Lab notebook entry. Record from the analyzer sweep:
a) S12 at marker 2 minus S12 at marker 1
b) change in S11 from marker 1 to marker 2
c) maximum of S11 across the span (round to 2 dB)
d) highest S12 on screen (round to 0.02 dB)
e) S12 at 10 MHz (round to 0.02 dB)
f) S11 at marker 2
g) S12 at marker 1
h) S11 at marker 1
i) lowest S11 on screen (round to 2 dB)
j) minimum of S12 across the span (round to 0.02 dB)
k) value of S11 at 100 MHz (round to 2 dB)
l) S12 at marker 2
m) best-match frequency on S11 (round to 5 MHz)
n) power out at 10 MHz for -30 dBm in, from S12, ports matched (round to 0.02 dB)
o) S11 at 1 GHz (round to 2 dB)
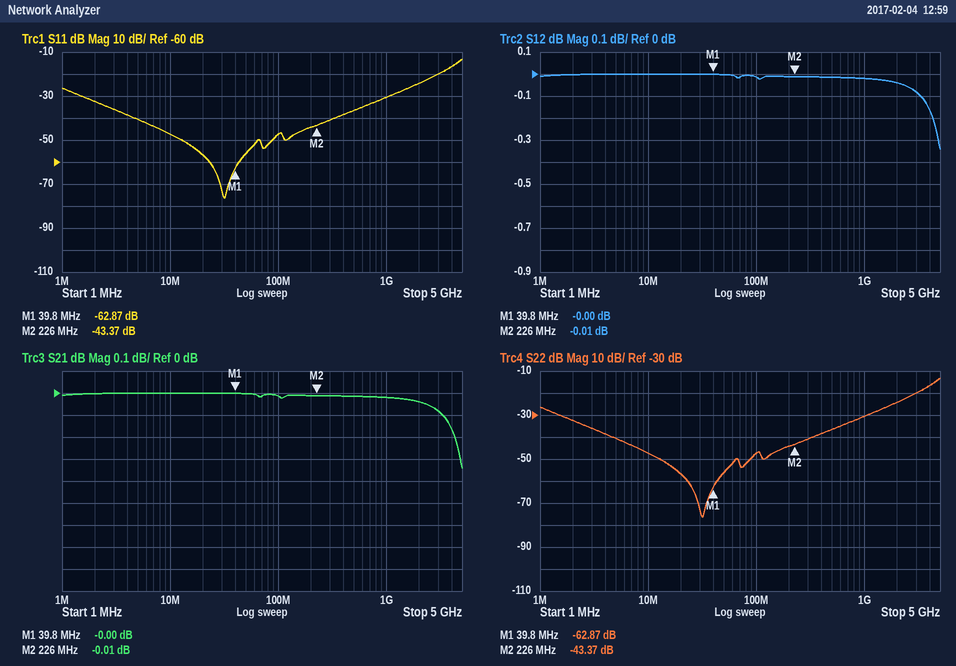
-0.01 dB
19.50 dB
-14 dB
0.00 dB
0.00 dB
-43.37 dB
-0.00 dB
-62.87 dB
-76 dB
-0.34 dB
-48 dB
-0.01 dB
30 MHz
-30.00 dBm
-30 dB
